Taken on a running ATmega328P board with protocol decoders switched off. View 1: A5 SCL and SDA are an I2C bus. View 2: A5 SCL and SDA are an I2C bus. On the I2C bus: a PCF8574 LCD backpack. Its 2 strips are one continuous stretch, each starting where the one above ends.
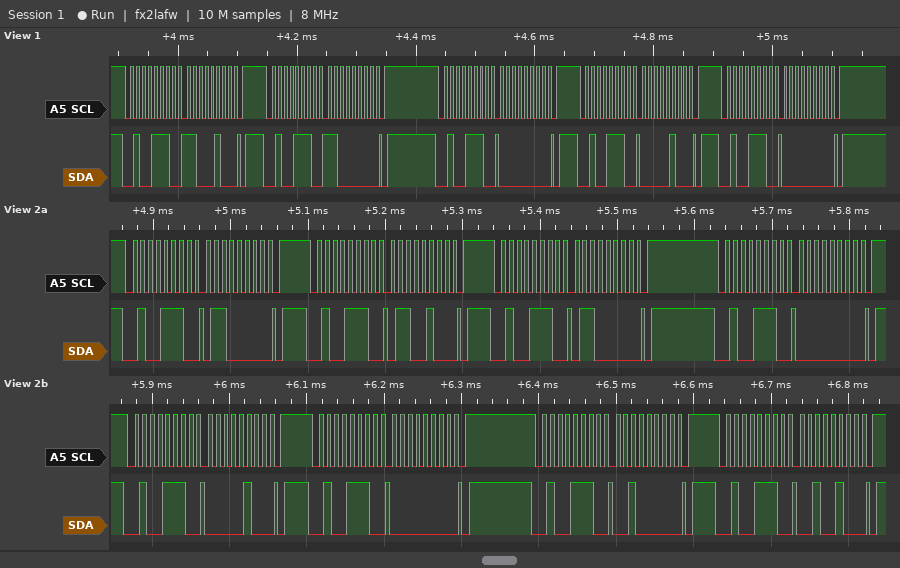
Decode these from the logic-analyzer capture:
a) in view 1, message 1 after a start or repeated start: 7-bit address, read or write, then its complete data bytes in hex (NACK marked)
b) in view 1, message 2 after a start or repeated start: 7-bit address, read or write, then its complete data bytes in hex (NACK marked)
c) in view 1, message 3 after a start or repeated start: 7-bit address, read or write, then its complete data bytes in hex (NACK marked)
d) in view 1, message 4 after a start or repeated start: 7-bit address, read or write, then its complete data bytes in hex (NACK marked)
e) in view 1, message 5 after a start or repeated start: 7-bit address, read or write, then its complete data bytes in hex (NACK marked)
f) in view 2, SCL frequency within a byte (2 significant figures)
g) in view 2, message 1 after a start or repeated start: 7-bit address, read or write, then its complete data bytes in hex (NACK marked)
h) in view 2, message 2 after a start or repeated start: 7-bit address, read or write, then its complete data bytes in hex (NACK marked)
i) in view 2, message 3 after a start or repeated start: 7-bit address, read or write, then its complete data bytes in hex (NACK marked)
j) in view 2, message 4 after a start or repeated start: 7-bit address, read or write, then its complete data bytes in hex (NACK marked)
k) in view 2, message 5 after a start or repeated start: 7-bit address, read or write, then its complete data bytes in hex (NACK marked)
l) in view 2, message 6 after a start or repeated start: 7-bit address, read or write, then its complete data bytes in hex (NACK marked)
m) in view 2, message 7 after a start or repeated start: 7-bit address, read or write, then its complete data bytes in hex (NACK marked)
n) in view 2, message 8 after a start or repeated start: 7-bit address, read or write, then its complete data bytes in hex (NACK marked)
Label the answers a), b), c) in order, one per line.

a) 0x27 write: C4
b) 0x27 write: C0
c) 0x27 write: 00
d) 0x27 write: 04
e) 0x27 write: 00
f) 100 kHz
g) 0x27 write: 60
h) 0x27 write: 64
i) 0x27 write: 60
j) 0x27 write: 00
k) 0x27 write: 04
l) 0x27 write: 00
m) 0x27 write: 20
n) 0x27 write: 24
